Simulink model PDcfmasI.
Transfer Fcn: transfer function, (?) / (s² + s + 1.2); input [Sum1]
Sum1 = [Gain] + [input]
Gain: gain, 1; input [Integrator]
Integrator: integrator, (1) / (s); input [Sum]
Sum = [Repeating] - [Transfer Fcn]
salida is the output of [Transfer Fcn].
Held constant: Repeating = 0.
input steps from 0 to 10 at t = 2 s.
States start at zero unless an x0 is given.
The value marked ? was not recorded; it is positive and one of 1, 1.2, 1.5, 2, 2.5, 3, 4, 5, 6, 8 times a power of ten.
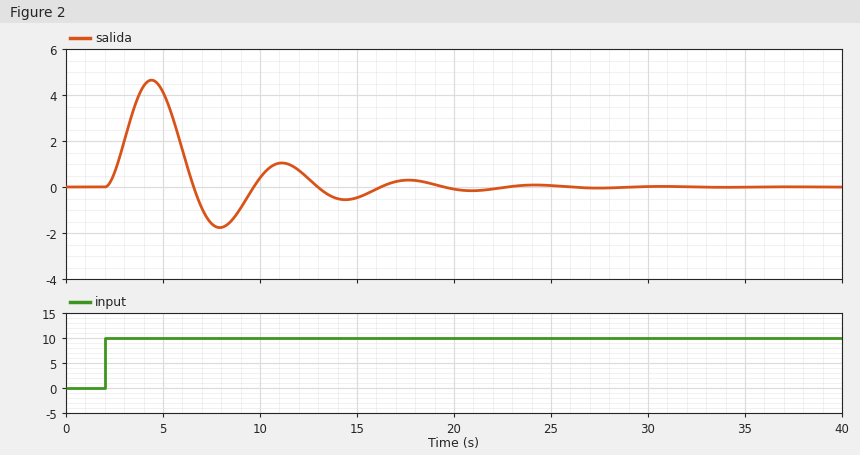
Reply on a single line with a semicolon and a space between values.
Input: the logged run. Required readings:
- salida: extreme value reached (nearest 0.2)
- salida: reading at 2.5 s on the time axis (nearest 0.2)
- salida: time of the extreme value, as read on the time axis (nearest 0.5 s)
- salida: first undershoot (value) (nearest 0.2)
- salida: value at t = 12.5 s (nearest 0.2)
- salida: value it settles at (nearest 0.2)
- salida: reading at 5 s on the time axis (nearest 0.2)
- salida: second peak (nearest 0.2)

4.6; 0.6; 4.5 s; -1.8; 0.4; 0.0; 4.2; 1.0
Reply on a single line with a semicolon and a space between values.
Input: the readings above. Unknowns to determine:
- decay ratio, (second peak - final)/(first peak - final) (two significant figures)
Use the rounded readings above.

0.22
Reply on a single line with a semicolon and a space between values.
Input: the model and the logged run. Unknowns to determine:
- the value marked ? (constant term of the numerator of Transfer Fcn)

0.6
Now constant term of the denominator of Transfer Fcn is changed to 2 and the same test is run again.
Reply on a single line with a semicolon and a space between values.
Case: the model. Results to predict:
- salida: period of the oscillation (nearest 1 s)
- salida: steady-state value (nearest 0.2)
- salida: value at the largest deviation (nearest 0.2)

5 s; 0.0; 3.4
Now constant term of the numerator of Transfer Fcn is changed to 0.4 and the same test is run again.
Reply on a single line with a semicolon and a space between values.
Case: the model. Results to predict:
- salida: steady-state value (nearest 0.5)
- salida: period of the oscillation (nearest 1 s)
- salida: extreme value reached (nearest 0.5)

0.0; 7 s; 3.5
